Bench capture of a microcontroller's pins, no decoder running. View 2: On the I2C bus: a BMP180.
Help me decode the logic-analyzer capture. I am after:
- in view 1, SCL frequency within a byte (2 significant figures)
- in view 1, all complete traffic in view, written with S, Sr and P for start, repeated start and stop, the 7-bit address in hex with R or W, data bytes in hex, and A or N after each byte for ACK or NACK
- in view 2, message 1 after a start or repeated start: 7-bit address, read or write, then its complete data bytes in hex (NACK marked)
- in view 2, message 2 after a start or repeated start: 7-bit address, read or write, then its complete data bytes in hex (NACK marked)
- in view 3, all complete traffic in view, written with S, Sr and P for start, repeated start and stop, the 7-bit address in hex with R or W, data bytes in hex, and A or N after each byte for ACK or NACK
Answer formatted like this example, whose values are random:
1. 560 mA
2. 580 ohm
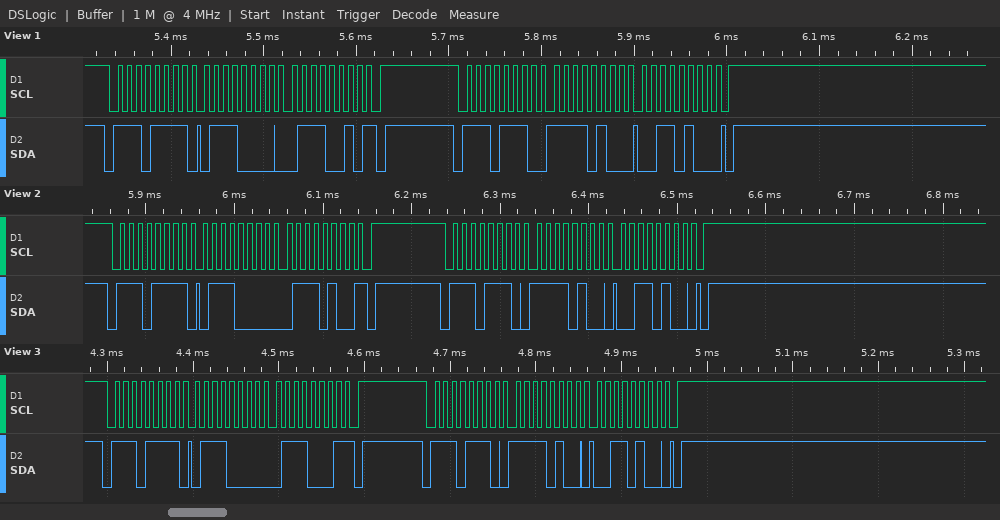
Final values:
1. 100 kHz
2. S 77R A 70 A 72 N P S 77W A F4 A 34 A P
3. 0x77 read: 70 74 NACK
4. 0x77 write: F4 34
5. S 77R A 70 A 71 N P S 77W A F4 A 34 A P
